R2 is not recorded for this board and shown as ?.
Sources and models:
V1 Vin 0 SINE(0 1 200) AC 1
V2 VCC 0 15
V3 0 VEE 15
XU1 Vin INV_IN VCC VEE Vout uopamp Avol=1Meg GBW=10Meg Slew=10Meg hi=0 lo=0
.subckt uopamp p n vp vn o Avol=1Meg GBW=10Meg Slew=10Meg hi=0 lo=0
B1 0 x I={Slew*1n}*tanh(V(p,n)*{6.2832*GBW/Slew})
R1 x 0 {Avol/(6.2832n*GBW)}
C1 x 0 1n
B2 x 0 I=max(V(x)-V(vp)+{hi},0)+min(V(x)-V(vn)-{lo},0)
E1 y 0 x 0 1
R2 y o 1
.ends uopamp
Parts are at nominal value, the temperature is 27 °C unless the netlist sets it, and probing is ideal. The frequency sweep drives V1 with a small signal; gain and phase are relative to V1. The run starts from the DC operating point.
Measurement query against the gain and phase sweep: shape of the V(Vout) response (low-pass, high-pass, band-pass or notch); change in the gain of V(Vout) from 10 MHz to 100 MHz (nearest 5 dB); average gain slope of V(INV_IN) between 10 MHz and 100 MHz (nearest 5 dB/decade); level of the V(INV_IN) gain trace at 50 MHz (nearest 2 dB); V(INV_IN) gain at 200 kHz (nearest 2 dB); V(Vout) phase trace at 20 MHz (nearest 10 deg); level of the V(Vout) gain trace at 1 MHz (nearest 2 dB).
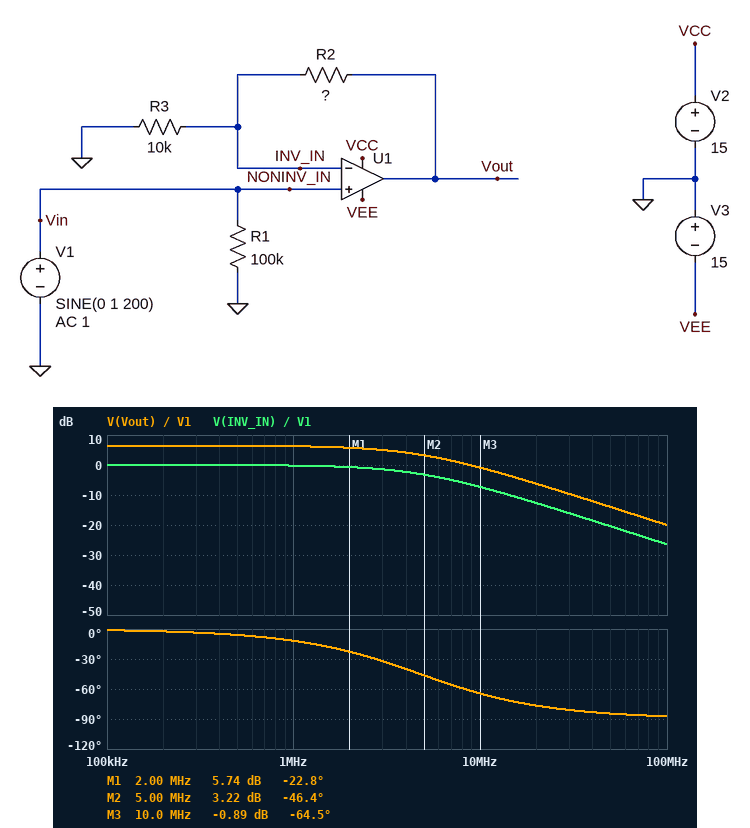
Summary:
low-pass
-20 dB
-20 dB/decade
-20 dB
0 dB
-80 deg
6 dB
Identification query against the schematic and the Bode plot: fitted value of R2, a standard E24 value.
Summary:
11 kΩ
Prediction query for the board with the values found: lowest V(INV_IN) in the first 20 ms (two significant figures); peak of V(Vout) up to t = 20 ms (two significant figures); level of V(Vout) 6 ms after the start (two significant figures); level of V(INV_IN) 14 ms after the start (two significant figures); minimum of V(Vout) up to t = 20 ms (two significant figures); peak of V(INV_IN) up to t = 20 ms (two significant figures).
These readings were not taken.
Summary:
-1.0 V
2.1 V
2.0 V
-950 mV
-2.1 V
1.0 V
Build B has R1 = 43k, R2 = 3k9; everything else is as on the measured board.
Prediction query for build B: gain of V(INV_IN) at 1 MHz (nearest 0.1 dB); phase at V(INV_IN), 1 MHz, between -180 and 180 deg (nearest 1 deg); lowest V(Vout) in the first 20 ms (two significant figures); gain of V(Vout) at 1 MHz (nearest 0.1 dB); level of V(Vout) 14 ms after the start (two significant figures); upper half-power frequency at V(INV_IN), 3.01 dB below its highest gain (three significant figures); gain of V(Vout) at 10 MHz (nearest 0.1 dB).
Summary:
-0.1 dB
-8 deg
-1.4 V
2.8 dB
-1.3 V
7.19 MHz
-1.8 dB
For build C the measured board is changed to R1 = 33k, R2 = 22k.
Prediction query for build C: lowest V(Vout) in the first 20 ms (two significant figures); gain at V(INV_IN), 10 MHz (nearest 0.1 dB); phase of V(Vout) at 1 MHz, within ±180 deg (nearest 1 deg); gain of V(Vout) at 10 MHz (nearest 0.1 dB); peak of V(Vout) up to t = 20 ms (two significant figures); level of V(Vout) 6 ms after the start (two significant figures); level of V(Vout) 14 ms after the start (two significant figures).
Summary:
-3.2 V
-10.5 dB
-18 deg
-0.4 dB
3.2 V
3.0 V
-3.0 V
